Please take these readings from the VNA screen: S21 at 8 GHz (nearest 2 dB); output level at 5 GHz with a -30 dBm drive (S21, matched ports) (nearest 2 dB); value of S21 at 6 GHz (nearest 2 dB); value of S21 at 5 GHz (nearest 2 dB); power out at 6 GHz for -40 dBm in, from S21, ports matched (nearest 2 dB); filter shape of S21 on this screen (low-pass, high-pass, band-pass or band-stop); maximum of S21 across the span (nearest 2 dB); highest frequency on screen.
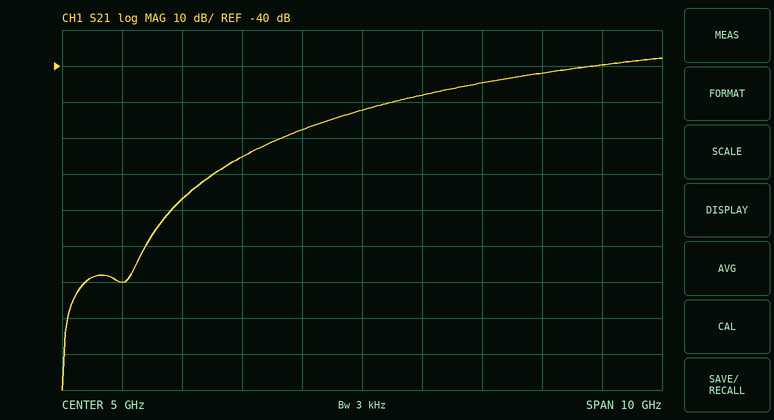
-42 dB
-82 dBm
-48 dB
-52 dB
-88 dBm
high-pass
-38 dB
10 GHz
